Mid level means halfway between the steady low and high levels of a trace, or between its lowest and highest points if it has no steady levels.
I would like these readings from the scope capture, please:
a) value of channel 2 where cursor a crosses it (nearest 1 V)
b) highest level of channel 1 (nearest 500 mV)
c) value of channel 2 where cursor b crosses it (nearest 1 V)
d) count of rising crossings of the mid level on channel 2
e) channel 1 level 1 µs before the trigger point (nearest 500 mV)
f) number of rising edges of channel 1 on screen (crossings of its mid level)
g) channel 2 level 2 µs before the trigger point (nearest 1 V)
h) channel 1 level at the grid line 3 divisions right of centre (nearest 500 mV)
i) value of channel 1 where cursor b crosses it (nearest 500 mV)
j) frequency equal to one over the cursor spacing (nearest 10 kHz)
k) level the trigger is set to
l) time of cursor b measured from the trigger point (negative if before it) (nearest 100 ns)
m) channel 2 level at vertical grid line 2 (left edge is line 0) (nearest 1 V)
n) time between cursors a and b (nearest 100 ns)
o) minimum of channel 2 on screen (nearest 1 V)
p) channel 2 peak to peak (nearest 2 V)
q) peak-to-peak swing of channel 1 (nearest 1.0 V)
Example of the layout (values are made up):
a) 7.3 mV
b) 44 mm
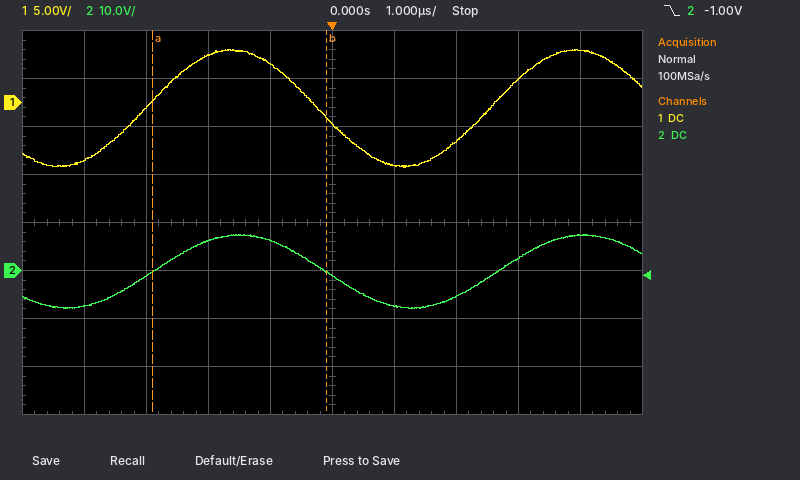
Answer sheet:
a) 0 V
b) 5.5 V
c) 0 V
d) 2
e) 4.0 V
f) 2
g) 6 V
h) 2.5 V
i) -1.5 V
j) 360 kHz
k) -1.00 V
l) -100 ns
m) -1 V
n) 2.8 µs
o) -8 V
p) 16 V
q) 12.0 V
